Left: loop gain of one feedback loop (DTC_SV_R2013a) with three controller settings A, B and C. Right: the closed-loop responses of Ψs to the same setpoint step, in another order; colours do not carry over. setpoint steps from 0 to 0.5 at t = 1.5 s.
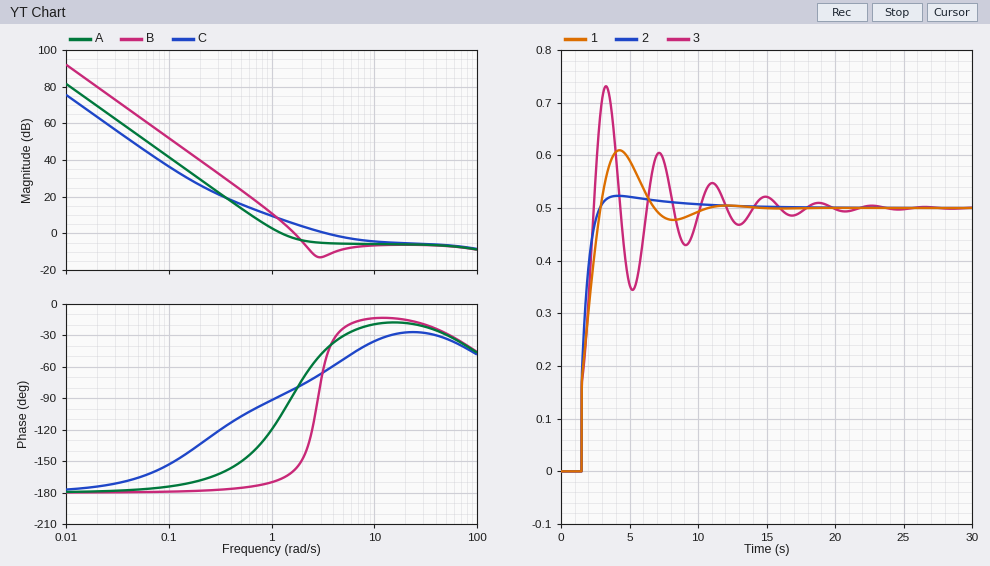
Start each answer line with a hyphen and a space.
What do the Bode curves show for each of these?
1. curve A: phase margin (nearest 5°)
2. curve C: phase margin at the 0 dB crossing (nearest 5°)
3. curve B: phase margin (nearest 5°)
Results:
- 75°
- 115°
- 20°
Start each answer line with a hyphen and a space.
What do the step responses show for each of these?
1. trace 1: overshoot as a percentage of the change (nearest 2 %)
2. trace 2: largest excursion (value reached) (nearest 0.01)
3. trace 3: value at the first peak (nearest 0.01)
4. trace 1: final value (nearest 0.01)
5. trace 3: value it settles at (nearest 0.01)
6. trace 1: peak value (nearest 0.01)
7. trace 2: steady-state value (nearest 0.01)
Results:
- 22 %
- 0.52
- 0.73
- 0.50
- 0.50
- 0.61
- 0.50
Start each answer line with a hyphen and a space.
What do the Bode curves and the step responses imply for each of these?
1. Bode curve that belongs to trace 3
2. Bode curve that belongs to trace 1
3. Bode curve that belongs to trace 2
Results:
- B
- A
- C
